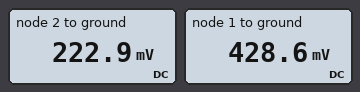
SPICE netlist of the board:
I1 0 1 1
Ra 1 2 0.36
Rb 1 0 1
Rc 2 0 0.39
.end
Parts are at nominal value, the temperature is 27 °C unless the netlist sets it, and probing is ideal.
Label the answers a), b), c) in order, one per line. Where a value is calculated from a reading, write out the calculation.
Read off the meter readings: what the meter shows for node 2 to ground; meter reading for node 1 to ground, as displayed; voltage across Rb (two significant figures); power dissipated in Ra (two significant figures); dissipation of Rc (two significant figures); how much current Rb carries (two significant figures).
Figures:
a) 222.9 mV
b) 428.6 mV
c) 428.6 mV = 430 mV
d) (428.6 mV - 222.9 mV)^2 / 360 mΩ = 120 mW
e) (222.9 mV)^2 / 390 mΩ = 130 mW
f) (428.6 mV) / 1 Ω = 430 mA
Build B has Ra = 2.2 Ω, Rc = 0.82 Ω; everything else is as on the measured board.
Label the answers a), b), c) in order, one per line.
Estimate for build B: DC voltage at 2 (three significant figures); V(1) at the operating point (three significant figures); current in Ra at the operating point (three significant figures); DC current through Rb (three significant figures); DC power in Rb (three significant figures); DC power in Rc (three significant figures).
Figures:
a) 204 mV
b) 751 mV
c) 249 mA
d) 751 mA
e) 564 mW
f) 50.7 mW
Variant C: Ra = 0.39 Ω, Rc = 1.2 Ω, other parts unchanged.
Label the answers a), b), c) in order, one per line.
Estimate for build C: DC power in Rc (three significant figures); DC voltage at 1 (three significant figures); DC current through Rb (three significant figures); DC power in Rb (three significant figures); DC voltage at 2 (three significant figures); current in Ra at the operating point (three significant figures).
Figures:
a) 179 mW
b) 614 mV
c) 614 mA
d) 377 mW
e) 463 mV
f) 386 mA
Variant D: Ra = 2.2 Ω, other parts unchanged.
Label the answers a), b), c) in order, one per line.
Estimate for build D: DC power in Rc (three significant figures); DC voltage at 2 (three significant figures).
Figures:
a) 30.3 mW
b) 109 mV
